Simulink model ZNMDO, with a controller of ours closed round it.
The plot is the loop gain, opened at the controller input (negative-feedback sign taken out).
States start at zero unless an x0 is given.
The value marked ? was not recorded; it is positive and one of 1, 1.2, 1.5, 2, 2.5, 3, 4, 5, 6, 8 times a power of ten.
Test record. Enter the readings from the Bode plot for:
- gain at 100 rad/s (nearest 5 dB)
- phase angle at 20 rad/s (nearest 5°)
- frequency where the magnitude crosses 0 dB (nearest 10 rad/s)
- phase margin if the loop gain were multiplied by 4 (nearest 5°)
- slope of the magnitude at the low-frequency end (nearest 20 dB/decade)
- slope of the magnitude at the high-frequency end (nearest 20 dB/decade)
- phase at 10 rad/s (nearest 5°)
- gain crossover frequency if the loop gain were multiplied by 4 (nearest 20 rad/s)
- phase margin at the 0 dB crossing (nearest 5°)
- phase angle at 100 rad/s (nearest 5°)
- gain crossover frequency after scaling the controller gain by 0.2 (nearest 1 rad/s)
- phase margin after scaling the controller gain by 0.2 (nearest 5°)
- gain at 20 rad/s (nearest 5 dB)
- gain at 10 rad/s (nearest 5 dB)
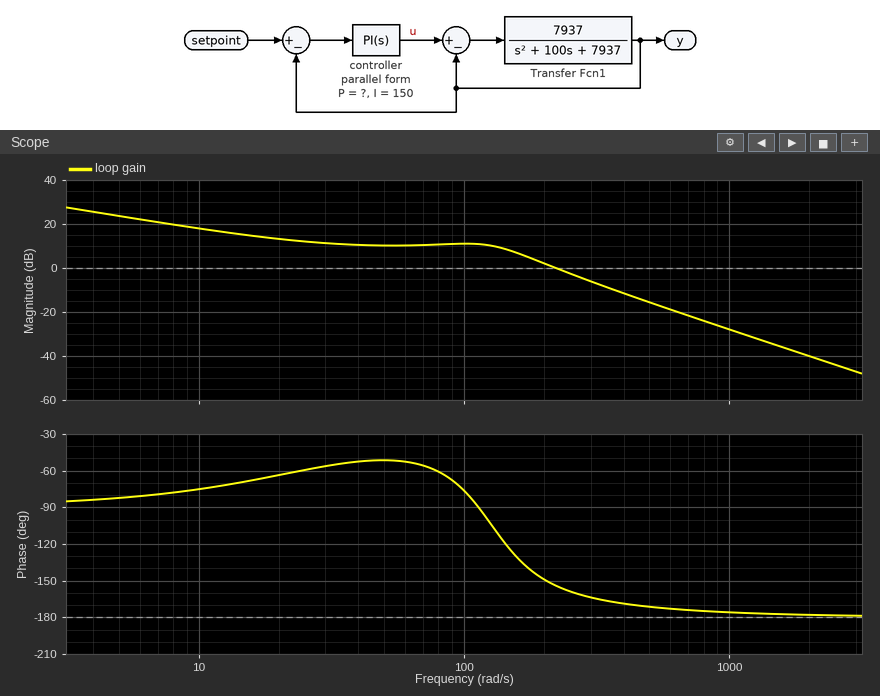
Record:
10 dB
-65°
220 rad/s
10°
-20 dB/decade
-40 dB/decade
-75°
420 rad/s
25°
-75°
18 rad/s
115°
15 dB
20 dB
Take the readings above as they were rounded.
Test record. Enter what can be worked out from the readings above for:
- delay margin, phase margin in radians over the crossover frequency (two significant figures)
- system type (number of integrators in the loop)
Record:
0.0020 s
1
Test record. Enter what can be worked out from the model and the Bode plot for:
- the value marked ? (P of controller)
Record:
5
